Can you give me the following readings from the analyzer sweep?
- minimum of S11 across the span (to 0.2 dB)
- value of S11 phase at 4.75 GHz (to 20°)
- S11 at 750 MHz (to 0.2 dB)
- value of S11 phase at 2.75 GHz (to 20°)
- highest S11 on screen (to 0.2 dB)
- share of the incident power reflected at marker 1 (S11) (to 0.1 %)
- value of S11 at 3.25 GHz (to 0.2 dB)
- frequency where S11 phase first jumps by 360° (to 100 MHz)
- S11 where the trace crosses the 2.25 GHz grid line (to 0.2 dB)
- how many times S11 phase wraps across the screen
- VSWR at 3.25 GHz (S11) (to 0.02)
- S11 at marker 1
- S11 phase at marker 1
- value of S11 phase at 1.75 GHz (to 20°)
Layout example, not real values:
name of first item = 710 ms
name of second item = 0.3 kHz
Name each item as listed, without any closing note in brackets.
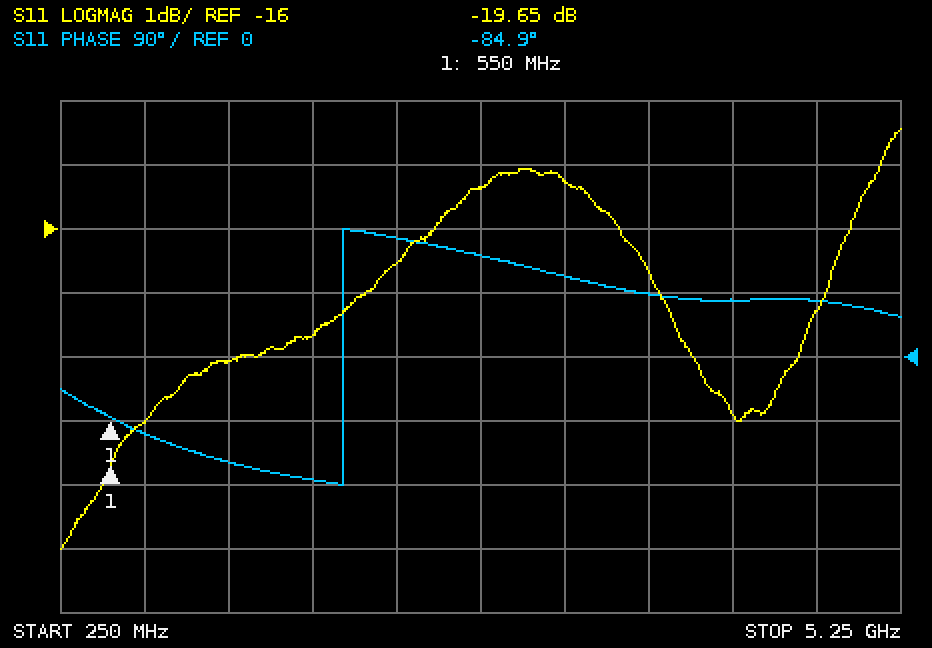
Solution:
minimum of S11 across the span = -21.0 dB
value of S11 phase at 4.75 GHz = 80°
S11 at 750 MHz = -19.0 dB
value of S11 phase at 2.75 GHz = 140°
highest S11 on screen = -14.4 dB
share of the incident power reflected at marker 1 (S11) = 1.1 %
value of S11 at 3.25 GHz = -15.2 dB
frequency where S11 phase first jumps by 360° = 1.9 GHz
S11 where the trace crosses the 2.25 GHz grid line = -16.6 dB
how many times S11 phase wraps across the screen = 1
VSWR at 3.25 GHz (S11) = 1.42
S11 at marker 1 = -19.65 dB
S11 phase at marker 1 = -84.9°
value of S11 phase at 1.75 GHz = -180°
